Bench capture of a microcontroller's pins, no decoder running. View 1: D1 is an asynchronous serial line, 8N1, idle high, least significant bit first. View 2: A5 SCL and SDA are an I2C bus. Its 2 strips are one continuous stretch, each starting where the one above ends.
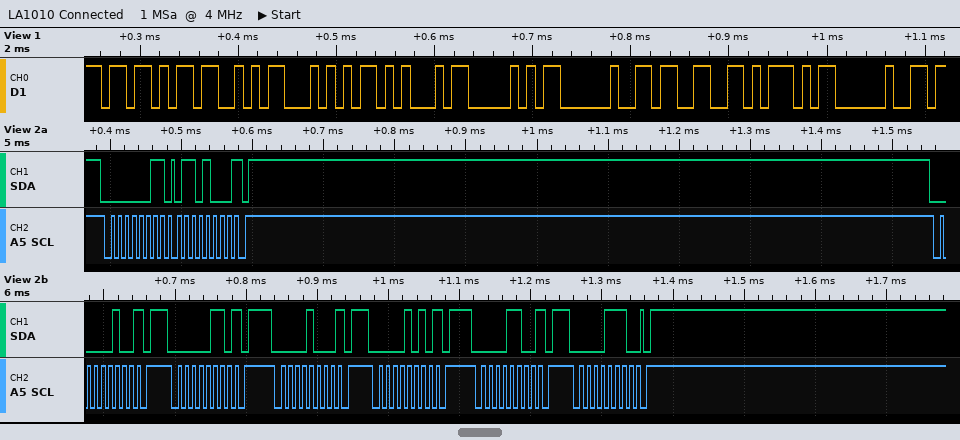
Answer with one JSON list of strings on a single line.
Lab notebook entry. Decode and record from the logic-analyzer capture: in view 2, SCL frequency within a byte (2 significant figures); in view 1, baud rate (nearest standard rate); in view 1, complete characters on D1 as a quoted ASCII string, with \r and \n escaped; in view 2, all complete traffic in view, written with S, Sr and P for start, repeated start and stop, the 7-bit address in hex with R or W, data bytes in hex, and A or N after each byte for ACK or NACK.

["100 kHz", "115200 baud", "\"[STEP 3] \"", "S 01R A 68 N P S 02W N P S 03W N P S 04W N P S 05W N P S 06W N P S 07W A P"]
